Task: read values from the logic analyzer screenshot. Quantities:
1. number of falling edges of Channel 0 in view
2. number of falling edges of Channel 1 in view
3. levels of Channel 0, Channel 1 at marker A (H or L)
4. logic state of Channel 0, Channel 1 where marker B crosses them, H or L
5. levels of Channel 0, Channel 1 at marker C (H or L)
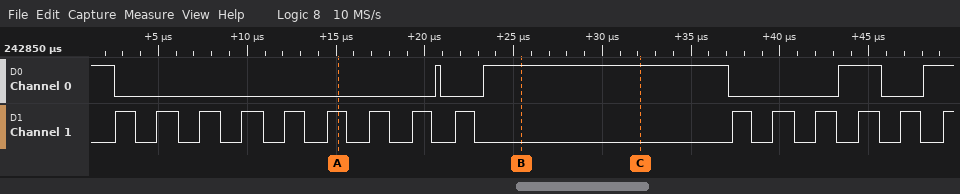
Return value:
4
14
Channel 0=L, Channel 1=H
Channel 0=H, Channel 1=L
Channel 0=H, Channel 1=L
